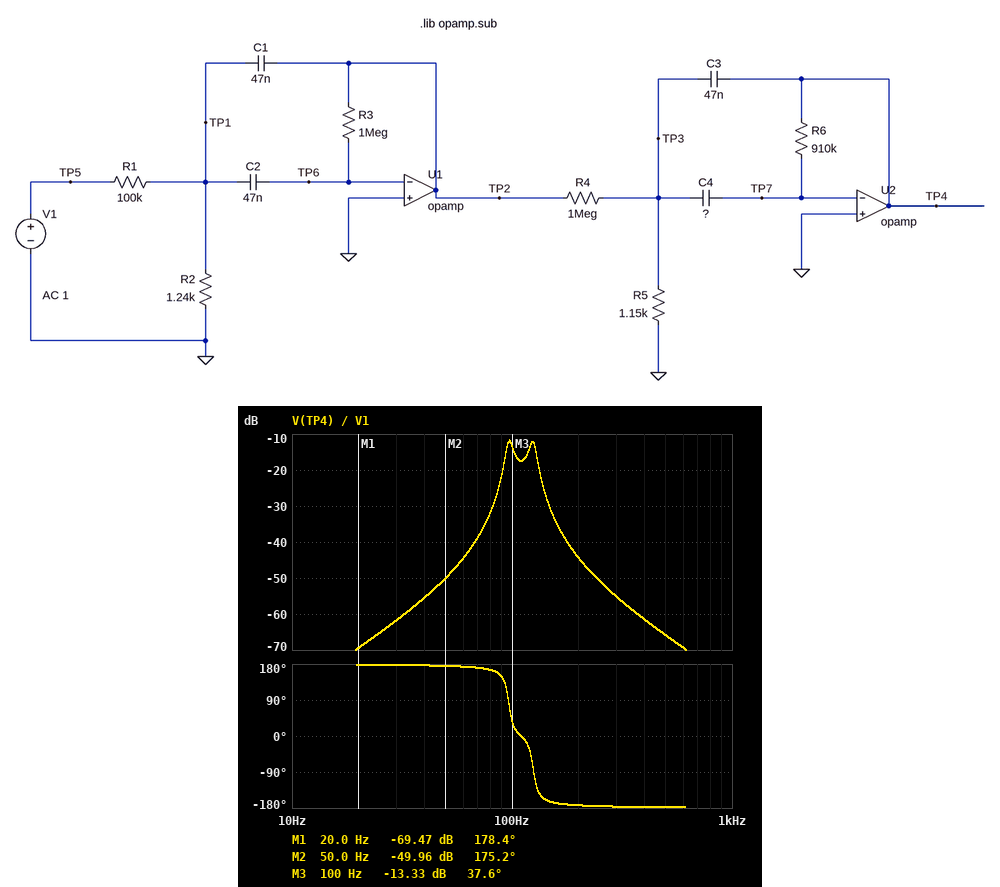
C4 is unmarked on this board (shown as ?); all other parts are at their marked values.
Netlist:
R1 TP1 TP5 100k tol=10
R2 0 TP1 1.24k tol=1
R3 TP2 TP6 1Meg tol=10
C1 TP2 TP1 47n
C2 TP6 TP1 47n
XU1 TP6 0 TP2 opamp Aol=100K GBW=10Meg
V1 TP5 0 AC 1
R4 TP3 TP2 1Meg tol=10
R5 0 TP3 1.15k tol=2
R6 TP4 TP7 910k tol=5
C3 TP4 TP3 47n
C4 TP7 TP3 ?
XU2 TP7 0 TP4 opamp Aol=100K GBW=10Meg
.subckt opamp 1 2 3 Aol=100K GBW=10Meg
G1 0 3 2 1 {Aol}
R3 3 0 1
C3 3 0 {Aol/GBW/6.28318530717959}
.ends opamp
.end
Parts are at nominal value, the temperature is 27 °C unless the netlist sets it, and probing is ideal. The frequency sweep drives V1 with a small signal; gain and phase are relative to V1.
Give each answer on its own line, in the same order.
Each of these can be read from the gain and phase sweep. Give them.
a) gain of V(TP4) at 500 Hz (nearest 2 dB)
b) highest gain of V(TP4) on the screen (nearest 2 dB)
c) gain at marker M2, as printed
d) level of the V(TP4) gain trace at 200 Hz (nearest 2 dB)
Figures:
-66 dB
-12 dB
-49.96 dB
-44 dB
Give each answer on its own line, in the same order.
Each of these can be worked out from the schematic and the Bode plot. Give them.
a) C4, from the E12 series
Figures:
33 nF
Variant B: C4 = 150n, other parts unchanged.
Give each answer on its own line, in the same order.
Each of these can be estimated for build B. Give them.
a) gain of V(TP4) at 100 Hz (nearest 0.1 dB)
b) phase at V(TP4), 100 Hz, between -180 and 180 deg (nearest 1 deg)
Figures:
-14.6 dB
-129 deg
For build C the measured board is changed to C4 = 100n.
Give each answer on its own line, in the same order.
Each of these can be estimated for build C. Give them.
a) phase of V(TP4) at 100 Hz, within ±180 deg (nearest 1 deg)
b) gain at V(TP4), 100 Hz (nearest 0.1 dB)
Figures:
-127 deg
-12.0 dB
